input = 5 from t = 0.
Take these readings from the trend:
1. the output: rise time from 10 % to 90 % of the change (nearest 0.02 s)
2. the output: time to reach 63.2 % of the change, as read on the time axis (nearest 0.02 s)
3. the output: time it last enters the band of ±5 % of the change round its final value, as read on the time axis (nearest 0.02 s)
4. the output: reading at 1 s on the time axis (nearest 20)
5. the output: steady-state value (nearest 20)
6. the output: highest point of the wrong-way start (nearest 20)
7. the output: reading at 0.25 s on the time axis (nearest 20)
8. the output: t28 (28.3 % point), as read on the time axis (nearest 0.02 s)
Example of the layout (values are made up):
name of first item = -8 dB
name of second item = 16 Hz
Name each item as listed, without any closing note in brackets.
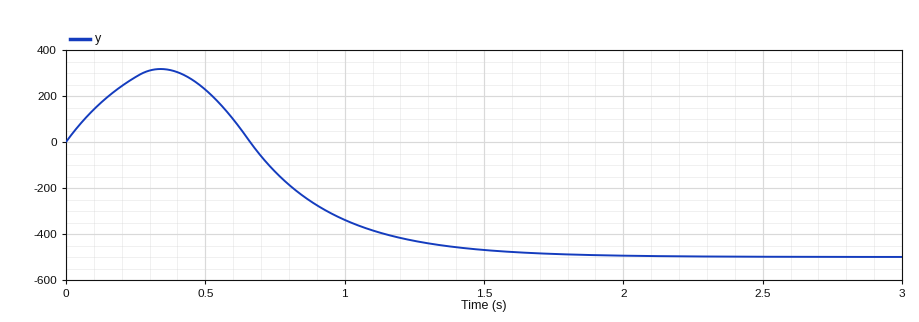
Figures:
the output: rise time from 10 % to 90 % of the change = 0.66 s
the output: time to reach 63.2 % of the change, as read on the time axis = 0.96 s
the output: time it last enters the band of ±5 % of the change round its final value, as read on the time axis = 1.56 s
the output: reading at 1 s on the time axis = -340
the output: steady-state value = -500
the output: highest point of the wrong-way start = 320
the output: reading at 0.25 s on the time axis = 280
the output: t28 (28.3 % point), as read on the time axis = 0.76 s
